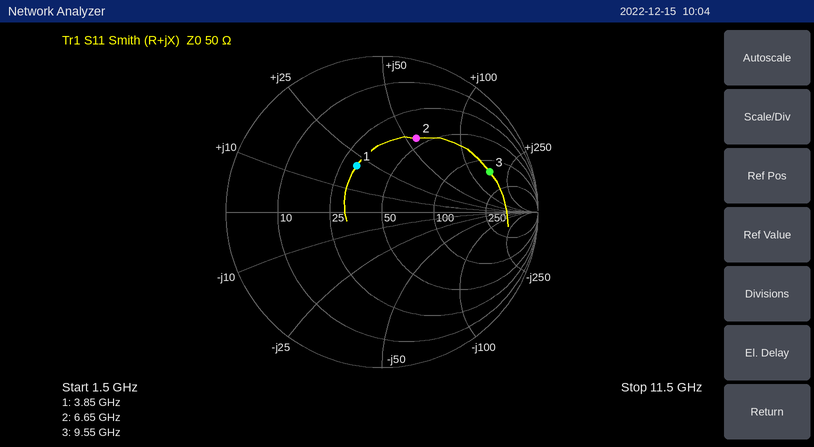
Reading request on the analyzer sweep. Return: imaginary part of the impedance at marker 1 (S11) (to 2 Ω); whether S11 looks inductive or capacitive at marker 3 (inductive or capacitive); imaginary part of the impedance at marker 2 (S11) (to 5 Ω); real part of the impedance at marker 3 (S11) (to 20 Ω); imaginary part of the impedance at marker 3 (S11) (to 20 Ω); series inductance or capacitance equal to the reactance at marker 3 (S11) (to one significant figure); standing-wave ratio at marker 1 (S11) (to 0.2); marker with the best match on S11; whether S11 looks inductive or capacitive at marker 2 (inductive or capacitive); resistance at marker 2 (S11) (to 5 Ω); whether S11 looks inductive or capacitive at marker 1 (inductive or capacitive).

+20 Ω
inductive
+55 Ω
140 Ω
+160 Ω
3 nH
2.0
marker 1
inductive
45 Ω
inductive
